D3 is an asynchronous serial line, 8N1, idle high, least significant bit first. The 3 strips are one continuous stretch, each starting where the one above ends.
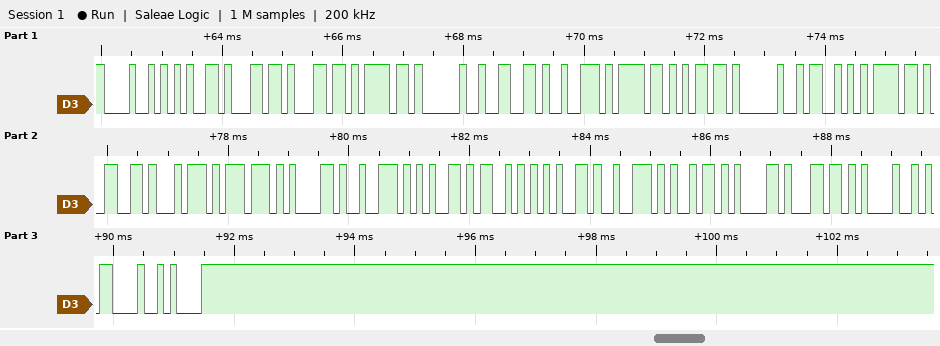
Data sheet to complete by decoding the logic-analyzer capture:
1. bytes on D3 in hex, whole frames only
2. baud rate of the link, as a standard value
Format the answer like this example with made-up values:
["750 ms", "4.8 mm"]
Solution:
["48 65 6C 6C 6F 20 66 72 6F 6D 20 53 6F 66 74 77 61 72 65 53 65 72 69 61 6C 21 0D 0A", "9600 baud"]
